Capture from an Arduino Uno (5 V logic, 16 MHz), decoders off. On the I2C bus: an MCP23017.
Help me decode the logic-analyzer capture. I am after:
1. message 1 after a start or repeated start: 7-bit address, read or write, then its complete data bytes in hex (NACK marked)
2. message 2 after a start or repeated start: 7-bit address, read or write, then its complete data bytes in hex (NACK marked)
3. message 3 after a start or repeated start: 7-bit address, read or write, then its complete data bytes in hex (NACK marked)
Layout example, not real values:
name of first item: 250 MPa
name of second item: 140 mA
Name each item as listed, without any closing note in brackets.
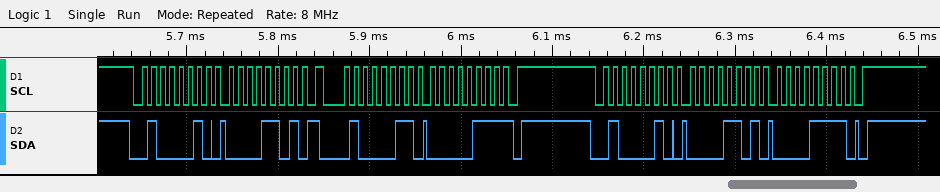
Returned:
message 1 after a start or repeated start: 7-bit address, read or write, then its complete data bytes in hex: 0x21 write: 0D
message 2 after a start or repeated start: 7-bit address, read or write, then its complete data bytes in hex: 0x21 read: 07 NACK
message 3 after a start or repeated start: 7-bit address, read or write, then its complete data bytes in hex: 0x21 write: 0D 0F
